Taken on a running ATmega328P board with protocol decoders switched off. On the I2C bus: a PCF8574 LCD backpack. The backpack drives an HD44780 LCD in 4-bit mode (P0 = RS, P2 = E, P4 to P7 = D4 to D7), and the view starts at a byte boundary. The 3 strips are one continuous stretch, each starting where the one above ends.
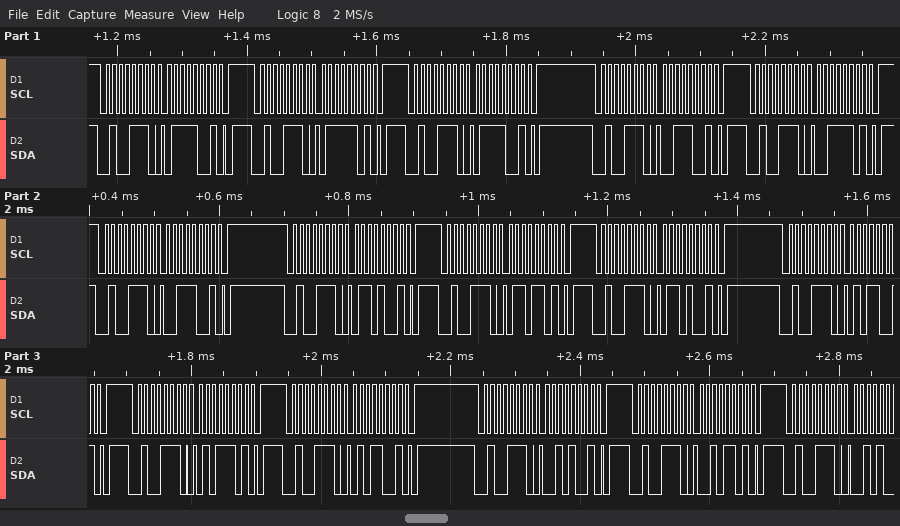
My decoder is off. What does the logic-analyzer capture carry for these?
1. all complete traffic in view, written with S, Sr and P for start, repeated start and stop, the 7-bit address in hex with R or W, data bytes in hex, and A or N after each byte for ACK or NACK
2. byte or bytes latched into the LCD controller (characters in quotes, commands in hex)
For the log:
S 27W A 79 A P S 27W A 7D A P S 27W A 79 A P S 27W A 39 A P S 27W A 3D A P S 27W A 39 A P S 27W A 69 A P S 27W A 6D A P S 27W A 69 A P S 27W A 59 A P S 27W A 5D A P S 27W A 59 A P S 27W A 29 A P S 27W A 2D A P S 27W A
's' 'e'
